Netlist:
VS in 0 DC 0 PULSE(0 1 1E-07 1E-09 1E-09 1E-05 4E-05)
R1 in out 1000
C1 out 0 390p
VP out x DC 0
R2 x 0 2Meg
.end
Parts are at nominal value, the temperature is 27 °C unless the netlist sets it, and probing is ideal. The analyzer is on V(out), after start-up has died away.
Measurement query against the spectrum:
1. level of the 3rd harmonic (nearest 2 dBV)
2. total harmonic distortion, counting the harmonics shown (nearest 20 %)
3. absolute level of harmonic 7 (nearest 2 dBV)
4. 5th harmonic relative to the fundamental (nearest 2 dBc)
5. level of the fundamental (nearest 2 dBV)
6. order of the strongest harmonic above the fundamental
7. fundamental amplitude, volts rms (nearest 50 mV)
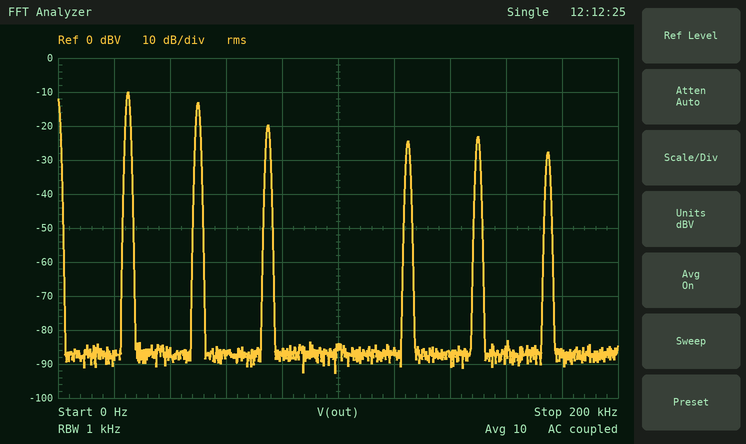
-20 dBV
80 %
-28 dBV
-14 dBc
-10 dBV
2
300 mV
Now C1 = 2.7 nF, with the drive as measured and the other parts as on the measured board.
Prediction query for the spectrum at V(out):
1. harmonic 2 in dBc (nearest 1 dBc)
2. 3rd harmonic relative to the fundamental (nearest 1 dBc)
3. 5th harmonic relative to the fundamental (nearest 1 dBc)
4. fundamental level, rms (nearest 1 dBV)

-5 dBc
-13 dBc
-21 dBc
-11 dBV
